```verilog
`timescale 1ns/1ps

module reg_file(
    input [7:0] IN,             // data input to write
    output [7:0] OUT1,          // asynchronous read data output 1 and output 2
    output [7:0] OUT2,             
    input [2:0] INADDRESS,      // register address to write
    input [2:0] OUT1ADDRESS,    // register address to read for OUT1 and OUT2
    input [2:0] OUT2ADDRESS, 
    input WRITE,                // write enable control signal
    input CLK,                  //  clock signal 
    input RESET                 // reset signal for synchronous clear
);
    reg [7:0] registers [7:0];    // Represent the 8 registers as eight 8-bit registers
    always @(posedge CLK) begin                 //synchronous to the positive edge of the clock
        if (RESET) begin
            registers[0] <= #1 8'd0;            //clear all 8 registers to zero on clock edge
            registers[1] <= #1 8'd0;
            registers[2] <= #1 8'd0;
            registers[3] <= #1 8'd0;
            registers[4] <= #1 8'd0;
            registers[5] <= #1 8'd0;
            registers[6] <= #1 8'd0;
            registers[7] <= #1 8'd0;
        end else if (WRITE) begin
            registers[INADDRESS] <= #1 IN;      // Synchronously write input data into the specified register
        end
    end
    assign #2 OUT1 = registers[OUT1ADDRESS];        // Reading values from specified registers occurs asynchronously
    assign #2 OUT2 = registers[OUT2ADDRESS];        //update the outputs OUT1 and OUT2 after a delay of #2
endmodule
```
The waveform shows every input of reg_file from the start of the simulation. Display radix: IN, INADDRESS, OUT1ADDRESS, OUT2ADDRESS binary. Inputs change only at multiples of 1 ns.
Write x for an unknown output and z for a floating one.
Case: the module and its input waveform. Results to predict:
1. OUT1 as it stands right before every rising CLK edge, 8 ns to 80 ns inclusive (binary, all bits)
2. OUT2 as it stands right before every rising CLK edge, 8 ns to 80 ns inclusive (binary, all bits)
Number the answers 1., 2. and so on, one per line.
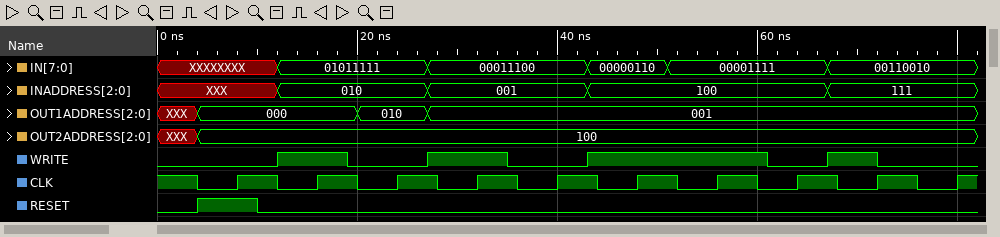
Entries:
1. x, 00000000, 01011111, 00000000, 00011100, 00011100, 00011100, 00011100, 00011100, 00011100
2. x, 00000000, 00000000, 00000000, 00000000, 00000000, 00000110, 00001111, 00001111, 00001111
